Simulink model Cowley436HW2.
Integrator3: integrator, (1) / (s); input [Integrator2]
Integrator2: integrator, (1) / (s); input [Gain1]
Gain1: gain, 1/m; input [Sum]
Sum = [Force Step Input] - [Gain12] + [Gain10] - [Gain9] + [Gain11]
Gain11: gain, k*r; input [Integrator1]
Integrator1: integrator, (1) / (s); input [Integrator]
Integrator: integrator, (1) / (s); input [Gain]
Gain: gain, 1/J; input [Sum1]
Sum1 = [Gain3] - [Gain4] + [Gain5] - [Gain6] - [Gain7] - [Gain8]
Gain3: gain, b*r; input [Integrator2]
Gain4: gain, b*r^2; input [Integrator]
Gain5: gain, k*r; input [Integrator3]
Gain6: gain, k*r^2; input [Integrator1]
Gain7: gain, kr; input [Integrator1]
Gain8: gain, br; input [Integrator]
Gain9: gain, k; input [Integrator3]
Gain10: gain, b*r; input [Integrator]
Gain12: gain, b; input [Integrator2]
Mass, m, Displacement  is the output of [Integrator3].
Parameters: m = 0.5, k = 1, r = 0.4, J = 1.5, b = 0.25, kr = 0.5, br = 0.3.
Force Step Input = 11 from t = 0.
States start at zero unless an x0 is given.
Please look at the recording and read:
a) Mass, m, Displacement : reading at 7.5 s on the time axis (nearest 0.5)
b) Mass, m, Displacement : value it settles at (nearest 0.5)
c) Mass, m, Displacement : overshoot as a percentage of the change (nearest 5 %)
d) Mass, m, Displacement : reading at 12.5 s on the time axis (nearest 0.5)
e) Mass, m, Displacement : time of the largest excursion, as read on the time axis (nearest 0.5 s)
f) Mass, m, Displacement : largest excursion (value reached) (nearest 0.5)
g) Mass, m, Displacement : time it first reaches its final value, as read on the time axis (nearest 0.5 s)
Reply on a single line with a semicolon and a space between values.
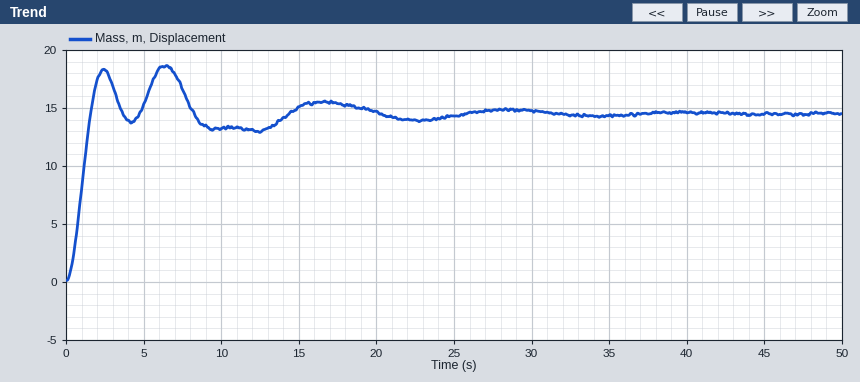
16.5; 14.5; 30 %; 13.0; 6.5 s; 18.5; 1.5 s
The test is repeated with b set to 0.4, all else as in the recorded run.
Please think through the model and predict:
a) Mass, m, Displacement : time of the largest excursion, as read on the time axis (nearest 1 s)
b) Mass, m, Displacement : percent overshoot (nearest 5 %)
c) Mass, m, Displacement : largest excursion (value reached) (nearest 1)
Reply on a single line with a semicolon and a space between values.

6 s; 20 %; 18
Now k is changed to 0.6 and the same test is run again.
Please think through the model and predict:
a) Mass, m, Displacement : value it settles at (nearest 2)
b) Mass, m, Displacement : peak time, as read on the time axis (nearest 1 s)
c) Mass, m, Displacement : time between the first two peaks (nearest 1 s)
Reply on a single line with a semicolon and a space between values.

22; 3 s; 5 s
